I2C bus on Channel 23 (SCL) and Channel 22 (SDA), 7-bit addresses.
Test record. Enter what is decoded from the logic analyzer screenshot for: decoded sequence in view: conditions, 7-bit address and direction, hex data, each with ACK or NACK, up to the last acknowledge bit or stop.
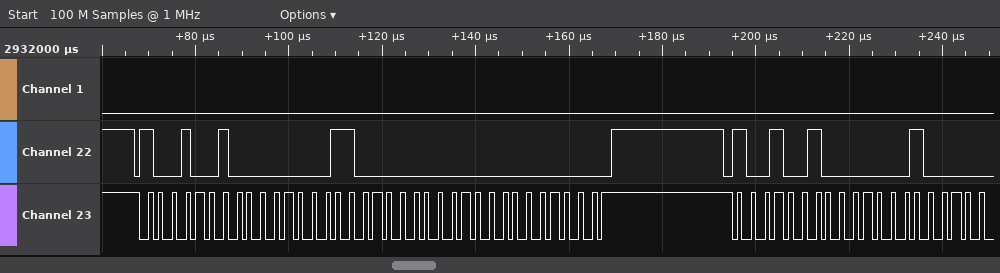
start, address 49 write ACK, 03 ACK, 00 ACK, 00 ACK, stop, start, address 49 write ACK, 04 ACK
